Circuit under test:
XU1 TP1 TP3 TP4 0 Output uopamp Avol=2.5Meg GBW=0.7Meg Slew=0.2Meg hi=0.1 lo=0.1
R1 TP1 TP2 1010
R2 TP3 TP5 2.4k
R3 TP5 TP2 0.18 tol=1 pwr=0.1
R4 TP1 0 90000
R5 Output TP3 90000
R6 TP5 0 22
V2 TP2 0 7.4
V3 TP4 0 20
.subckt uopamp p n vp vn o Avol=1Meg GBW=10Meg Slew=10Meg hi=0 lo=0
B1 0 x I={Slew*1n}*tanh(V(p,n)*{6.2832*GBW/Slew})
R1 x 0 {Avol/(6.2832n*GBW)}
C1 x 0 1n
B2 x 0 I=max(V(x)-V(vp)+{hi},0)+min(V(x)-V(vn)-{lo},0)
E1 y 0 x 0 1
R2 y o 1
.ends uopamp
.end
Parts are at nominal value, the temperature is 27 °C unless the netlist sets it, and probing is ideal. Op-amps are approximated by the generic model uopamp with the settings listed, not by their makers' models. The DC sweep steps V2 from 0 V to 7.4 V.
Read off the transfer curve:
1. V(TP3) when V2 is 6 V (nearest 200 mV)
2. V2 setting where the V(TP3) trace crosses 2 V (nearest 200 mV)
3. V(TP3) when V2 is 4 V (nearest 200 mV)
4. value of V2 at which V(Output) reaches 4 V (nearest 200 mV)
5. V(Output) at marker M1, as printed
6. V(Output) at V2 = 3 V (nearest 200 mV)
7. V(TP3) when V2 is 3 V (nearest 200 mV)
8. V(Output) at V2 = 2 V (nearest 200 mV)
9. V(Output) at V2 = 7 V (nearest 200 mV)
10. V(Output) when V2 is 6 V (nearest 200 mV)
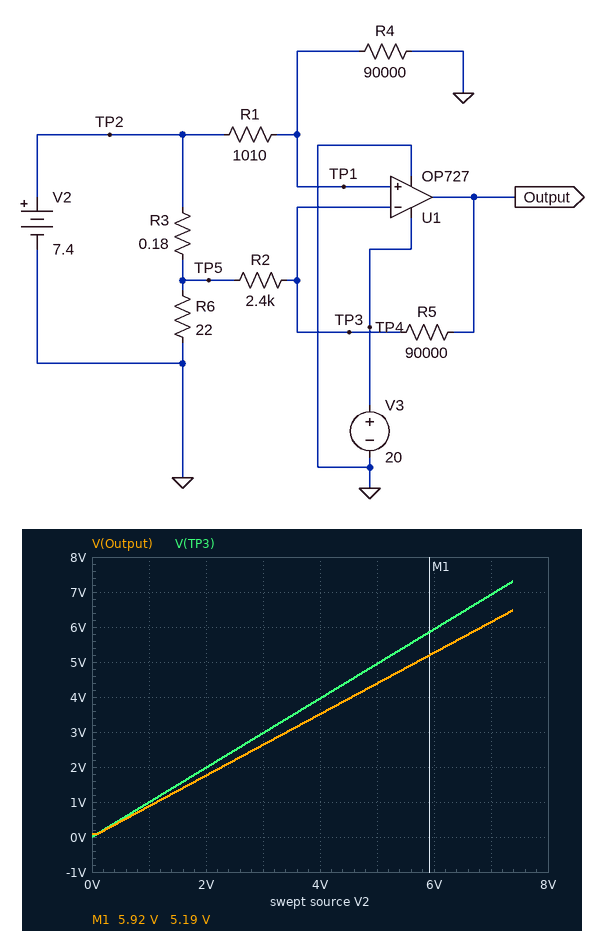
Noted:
6.0 V
2.0 V
4.0 V
4.6 V
5.19 V
2.6 V
3.0 V
1.8 V
6.2 V
5.2 V
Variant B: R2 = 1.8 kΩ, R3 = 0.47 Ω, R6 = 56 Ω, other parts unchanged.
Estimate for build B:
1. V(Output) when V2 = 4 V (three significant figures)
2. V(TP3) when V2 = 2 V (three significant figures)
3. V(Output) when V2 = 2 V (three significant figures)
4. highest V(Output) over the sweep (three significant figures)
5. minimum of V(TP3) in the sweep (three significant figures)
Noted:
3.40 V
1.98 V
1.70 V
6.29 V
1.96 mV
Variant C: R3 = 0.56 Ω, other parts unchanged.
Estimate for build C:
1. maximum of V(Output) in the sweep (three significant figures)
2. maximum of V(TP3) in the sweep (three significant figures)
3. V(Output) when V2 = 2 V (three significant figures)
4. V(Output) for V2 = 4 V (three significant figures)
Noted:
11.1 V
7.32 V
3.01 V
6.01 V
